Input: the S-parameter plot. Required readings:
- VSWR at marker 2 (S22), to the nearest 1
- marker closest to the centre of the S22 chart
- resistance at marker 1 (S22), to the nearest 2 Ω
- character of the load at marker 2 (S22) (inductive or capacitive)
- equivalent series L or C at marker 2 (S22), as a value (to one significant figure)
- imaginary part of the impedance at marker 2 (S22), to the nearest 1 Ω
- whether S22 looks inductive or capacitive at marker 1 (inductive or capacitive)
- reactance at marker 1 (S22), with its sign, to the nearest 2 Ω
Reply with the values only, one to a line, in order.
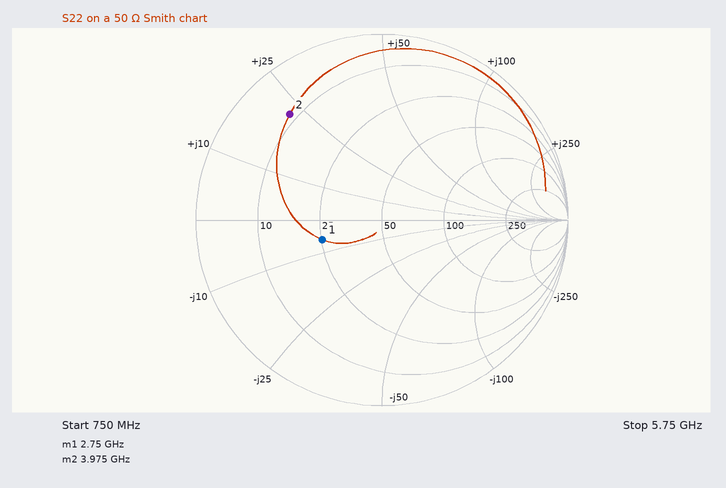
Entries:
7
marker 1
26 Ω
inductive
900 pH
+22 Ω
capacitive
-6 Ω
